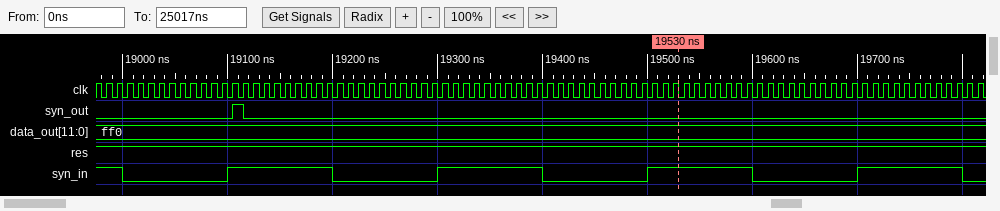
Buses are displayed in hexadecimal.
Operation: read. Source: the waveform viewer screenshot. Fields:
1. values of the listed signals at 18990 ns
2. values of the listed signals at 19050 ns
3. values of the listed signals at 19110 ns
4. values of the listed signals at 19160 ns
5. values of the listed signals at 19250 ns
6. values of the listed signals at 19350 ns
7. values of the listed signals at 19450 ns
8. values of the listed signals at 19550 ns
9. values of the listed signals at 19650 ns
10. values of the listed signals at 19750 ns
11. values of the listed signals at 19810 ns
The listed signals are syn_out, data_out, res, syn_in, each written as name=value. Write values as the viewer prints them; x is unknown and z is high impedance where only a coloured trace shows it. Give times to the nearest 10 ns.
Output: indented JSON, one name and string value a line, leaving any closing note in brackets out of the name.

{
  "values of the listed signals at 18990 ns": "syn_out=0, data_out=ff0, res=1, syn_in=1",
  "values of the listed signals at 19050 ns": "syn_out=0, data_out=ff0, res=1, syn_in=0",
  "values of the listed signals at 19110 ns": "syn_out=1, data_out=ff0, res=1, syn_in=1",
  "values of the listed signals at 19160 ns": "syn_out=0, data_out=ff0, res=1, syn_in=1",
  "values of the listed signals at 19250 ns": "syn_out=0, data_out=ff0, res=1, syn_in=0",
  "values of the listed signals at 19350 ns": "syn_out=0, data_out=ff0, res=1, syn_in=1",
  "values of the listed signals at 19450 ns": "syn_out=0, data_out=ff0, res=1, syn_in=0",
  "values of the listed signals at 19550 ns": "syn_out=0, data_out=ff0, res=1, syn_in=1",
  "values of the listed signals at 19650 ns": "syn_out=0, data_out=ff0, res=1, syn_in=0",
  "values of the listed signals at 19750 ns": "syn_out=0, data_out=ff0, res=1, syn_in=1",
  "values of the listed signals at 19810 ns": "syn_out=0, data_out=ff0, res=1, syn_in=0"
}
